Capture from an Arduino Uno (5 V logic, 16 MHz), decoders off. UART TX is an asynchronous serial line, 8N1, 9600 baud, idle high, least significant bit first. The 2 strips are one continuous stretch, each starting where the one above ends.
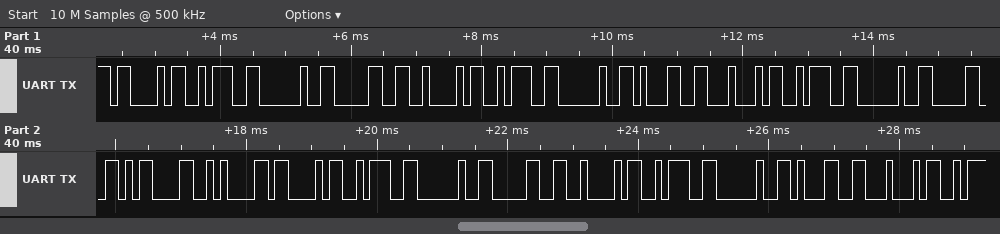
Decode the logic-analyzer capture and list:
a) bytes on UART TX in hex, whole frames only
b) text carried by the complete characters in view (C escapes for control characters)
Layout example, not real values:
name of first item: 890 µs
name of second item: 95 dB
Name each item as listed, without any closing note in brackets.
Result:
bytes on UART TX in hex, whole frames only: 43 3A 20 30 42 3A 20 31 44 3A 20 30 0D 0A 43 3A 20 30 42 3A 20 31 44
text carried by the complete characters in view: "C: 0B: 1D: 0\r\nC: 0B: 1D"
